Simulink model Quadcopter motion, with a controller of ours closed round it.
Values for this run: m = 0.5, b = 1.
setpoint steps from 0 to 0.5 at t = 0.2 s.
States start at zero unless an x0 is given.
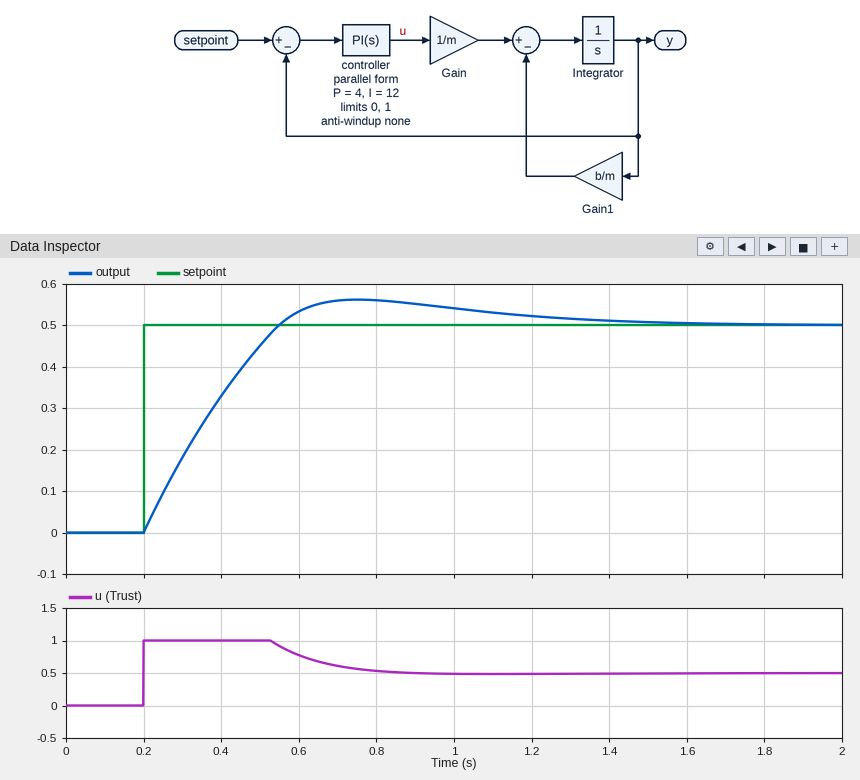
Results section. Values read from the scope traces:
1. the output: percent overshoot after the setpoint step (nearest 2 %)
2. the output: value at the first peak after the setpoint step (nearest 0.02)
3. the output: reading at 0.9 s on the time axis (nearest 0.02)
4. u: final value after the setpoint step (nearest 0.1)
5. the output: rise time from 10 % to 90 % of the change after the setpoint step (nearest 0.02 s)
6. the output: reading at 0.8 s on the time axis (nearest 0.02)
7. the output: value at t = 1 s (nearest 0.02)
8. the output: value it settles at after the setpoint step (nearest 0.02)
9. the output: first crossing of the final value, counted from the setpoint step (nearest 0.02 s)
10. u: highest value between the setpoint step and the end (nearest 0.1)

12 %
0.56
0.56
0.5
0.28 s
0.56
0.54
0.50
0.34 s
1.0
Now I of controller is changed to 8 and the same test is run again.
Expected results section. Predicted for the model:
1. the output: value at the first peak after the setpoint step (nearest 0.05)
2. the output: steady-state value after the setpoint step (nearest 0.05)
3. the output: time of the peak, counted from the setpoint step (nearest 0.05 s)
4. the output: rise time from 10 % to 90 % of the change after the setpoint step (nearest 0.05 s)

0.50
0.50
0.65 s
0.30 s
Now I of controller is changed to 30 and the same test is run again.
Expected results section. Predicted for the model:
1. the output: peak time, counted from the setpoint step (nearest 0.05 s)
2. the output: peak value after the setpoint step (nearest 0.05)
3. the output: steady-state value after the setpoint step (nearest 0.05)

0.60 s
0.70
0.50
